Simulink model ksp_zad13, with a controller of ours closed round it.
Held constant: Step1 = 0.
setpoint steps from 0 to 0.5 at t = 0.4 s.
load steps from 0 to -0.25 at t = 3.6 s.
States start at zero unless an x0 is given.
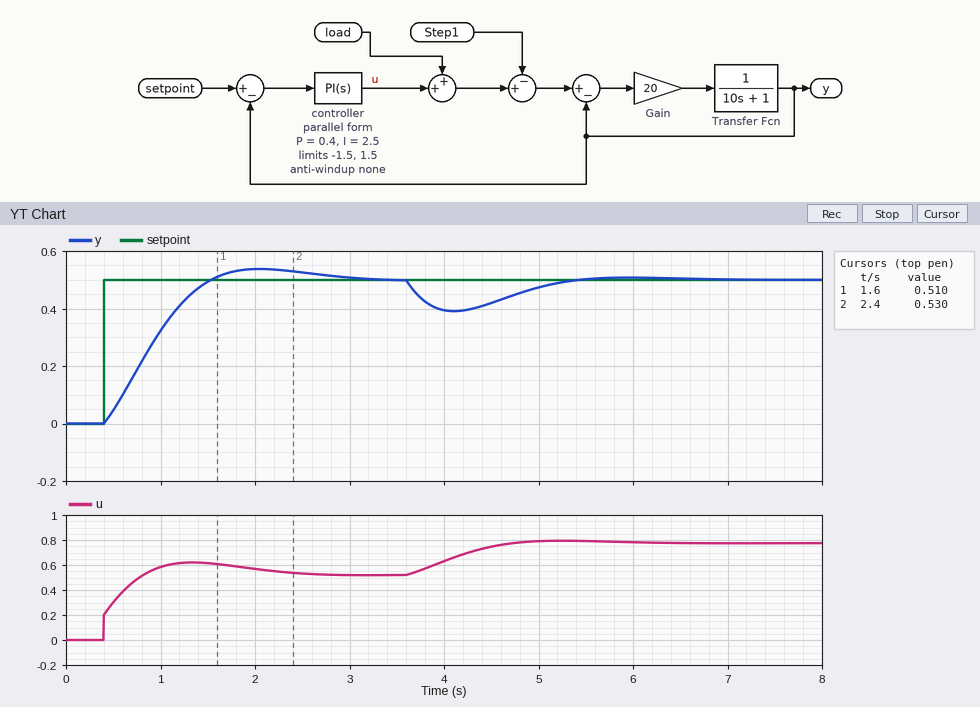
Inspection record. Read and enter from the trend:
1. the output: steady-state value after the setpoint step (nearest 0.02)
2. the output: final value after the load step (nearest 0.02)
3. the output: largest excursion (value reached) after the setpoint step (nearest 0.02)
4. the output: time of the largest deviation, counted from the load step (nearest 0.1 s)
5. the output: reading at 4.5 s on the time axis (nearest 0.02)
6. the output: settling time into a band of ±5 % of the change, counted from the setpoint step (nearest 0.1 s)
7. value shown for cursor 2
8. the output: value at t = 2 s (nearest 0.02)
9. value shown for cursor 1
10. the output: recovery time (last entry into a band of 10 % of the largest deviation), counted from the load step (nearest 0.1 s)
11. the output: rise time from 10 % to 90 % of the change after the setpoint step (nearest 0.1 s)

0.50
0.50
0.54
0.5 s
0.42
2.1 s
0.530
0.54
0.510
1.6 s
0.8 s
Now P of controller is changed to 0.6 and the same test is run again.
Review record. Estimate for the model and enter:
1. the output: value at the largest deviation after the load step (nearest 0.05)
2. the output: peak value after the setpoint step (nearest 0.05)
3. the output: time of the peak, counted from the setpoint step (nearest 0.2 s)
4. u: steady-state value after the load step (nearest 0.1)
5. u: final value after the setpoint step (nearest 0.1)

0.40
0.50
1.8 s
0.8
0.5
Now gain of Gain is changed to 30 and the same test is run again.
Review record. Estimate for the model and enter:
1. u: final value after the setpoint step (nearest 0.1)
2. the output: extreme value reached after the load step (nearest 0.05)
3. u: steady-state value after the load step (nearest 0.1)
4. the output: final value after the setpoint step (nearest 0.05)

0.5
0.40
0.8
0.50
